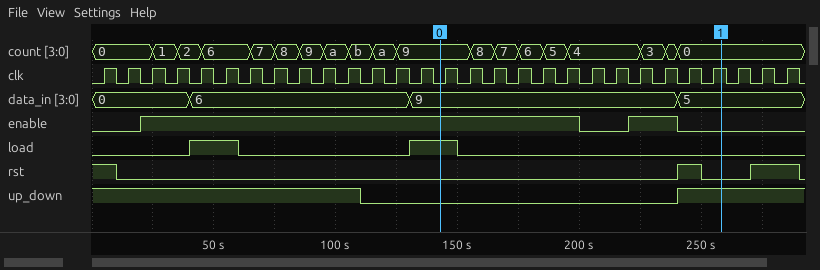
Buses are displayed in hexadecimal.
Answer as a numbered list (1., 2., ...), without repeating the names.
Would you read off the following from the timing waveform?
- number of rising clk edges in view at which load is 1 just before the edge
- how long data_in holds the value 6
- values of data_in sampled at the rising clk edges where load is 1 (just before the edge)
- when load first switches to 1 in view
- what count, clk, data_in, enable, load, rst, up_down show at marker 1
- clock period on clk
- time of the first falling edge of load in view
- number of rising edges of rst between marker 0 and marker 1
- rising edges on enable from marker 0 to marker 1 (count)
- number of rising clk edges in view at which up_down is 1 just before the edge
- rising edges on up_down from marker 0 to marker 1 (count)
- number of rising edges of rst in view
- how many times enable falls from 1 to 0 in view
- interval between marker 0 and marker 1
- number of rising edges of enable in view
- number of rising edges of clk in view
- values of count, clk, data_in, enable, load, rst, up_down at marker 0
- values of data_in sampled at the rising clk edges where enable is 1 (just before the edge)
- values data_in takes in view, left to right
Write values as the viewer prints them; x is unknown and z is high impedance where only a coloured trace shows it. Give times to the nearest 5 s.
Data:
1. 4
2. 90 s
3. 6, 6, 9, 9
4. 40 s
5. count=0, clk=1, data_in=5, enable=0, load=0, rst=0, up_down=1
6. 10 s
7. 60 s
8. 1
9. 1
10. 16
11. 1
12. 2
13. 2
14. 115 s
15. 2
16. 29
17. count=9, clk=0, data_in=9, enable=1, load=1, rst=0, up_down=0
18. 0, 0, 6, 6, 6, 6, 6, 6, 6, 6, 6, 9, 9, 9, 9, 9, 9, 9, 9, 9
19. 0, 6, 9, 5
